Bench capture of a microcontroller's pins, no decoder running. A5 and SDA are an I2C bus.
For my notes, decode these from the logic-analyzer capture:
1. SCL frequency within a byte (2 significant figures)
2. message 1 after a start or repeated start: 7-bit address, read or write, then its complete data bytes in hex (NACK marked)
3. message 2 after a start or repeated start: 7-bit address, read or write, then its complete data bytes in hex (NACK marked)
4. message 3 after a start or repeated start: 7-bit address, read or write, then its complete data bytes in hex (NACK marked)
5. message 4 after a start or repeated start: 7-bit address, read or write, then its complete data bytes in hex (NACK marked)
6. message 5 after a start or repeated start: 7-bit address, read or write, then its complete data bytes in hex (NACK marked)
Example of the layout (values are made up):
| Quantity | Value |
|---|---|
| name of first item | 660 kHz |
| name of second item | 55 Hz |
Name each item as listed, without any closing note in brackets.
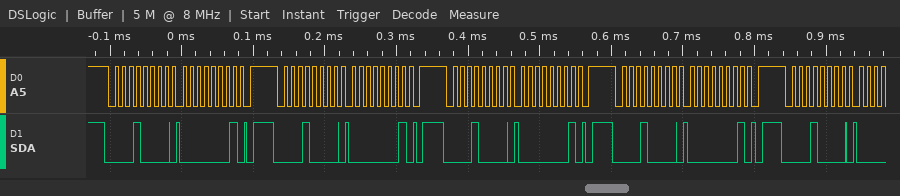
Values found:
| Quantity | Value |
|---|---|
| SCL frequency within a byte | 100 kHz |
| message 1 after a start or repeated start: 7-bit address, read or write, then its complete data bytes in hex | 0x08 write: 01 |
| message 2 after a start or repeated start: 7-bit address, read or write, then its complete data bytes in hex | 0x08 write: 01 |
| message 3 after a start or repeated start: 7-bit address, read or write, then its complete data bytes in hex | 0x08 write: 01 |
| message 4 after a start or repeated start: 7-bit address, read or write, then its complete data bytes in hex | 0x08 write: 01 |
| message 5 after a start or repeated start: 7-bit address, read or write, then its complete data bytes in hex | 0x08 write |
